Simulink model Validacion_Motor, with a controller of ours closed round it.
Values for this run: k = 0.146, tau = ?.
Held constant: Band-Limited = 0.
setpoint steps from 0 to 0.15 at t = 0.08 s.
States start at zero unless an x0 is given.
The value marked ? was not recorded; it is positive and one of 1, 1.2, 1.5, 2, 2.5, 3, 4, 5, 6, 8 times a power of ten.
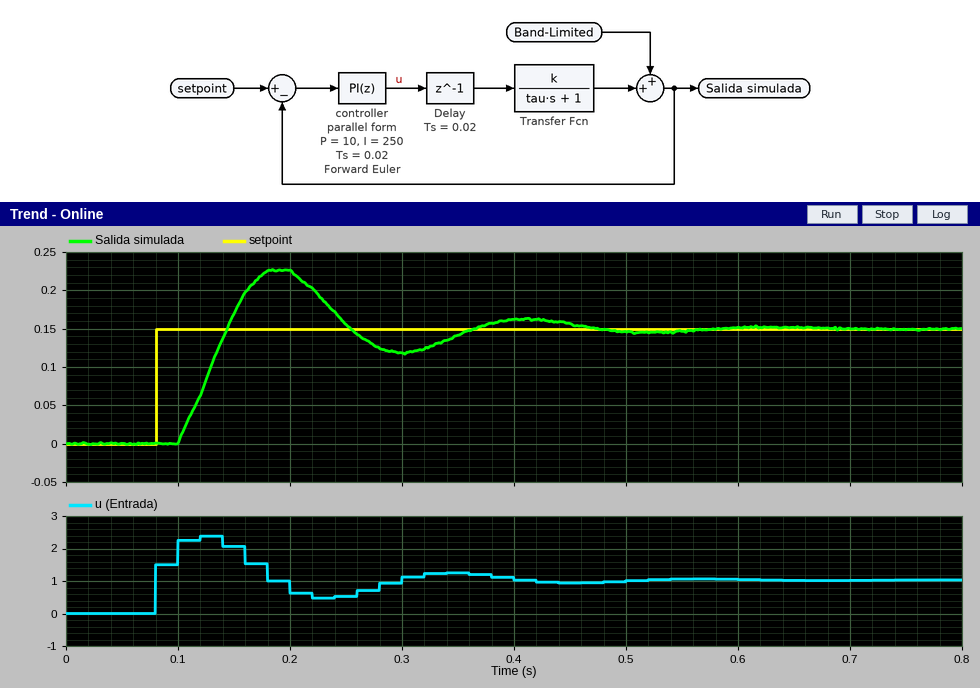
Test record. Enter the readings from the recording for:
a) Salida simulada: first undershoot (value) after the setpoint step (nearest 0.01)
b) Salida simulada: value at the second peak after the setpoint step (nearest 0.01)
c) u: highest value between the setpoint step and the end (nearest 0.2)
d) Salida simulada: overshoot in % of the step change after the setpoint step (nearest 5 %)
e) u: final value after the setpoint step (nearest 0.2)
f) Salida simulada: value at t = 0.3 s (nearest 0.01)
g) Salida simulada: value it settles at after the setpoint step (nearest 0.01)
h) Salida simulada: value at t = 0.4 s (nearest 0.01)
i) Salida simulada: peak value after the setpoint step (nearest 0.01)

0.12
0.16
2.4
50 %
1.0
0.12
0.15
0.16
0.23
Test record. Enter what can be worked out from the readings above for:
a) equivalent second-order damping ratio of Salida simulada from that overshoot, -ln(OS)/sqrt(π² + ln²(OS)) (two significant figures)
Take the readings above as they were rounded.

0.22
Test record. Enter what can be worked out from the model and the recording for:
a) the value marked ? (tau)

0.06
